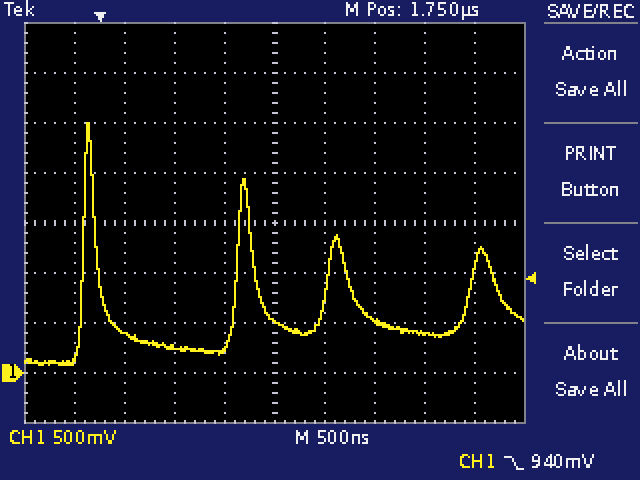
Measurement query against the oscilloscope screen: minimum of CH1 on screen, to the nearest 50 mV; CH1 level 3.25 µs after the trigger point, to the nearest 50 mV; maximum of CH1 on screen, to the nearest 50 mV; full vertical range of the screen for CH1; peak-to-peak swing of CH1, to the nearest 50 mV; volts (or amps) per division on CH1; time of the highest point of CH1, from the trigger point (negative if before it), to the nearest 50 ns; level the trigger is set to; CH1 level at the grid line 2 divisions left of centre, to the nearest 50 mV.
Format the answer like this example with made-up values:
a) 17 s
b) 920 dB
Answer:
a) 100 mV
b) 400 mV
c) 2.50 V
d) 4 V
e) 2.40 V
f) 500 mV
g) -100 ns
h) 940 mV
i) 250 mV
